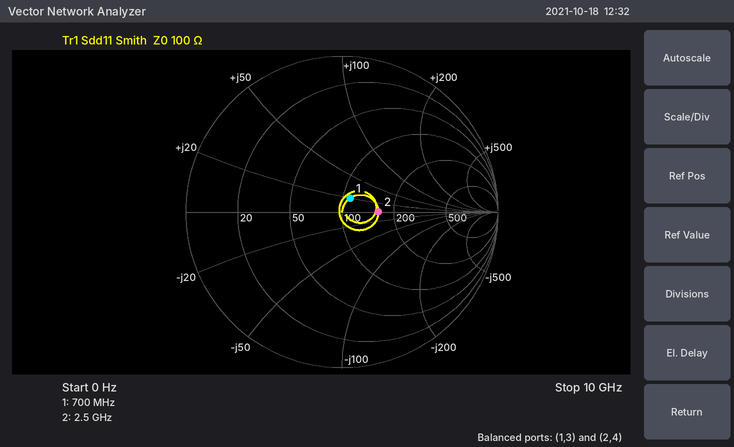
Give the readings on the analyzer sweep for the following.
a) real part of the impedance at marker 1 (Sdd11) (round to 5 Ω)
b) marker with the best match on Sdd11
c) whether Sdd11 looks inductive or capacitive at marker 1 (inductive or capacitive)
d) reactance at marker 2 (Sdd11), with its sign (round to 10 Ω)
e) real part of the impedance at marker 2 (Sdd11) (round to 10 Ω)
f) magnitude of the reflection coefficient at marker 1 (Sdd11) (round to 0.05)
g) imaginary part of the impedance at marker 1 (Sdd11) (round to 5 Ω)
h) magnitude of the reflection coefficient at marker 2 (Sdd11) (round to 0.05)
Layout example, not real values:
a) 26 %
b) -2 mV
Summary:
a) 110 Ω
b) marker 1
c) inductive
d) 0 Ω
e) 160 Ω
f) 0.10
g) +20 Ω
h) 0.25
